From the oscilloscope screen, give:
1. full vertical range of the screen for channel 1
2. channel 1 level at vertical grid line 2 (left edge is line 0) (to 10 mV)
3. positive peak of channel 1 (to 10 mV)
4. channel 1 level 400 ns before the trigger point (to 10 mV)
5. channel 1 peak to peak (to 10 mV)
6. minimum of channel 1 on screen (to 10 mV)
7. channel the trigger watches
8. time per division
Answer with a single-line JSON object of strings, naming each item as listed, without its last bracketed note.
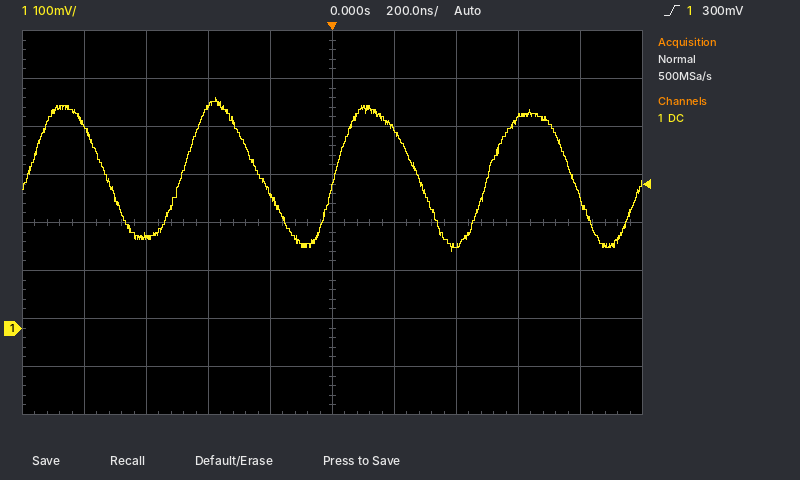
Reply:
{"full vertical range of the screen for channel 1": "800 mV", "channel 1 level at vertical grid line 2 (left edge is line 0)": "190 mV", "positive peak of channel 1": "480 mV", "channel 1 level 400 ns before the trigger point": "460 mV", "channel 1 peak to peak": "320 mV", "minimum of channel 1 on screen": "160 mV", "channel the trigger watches": "channel 1", "time per division": "200 ns"}
